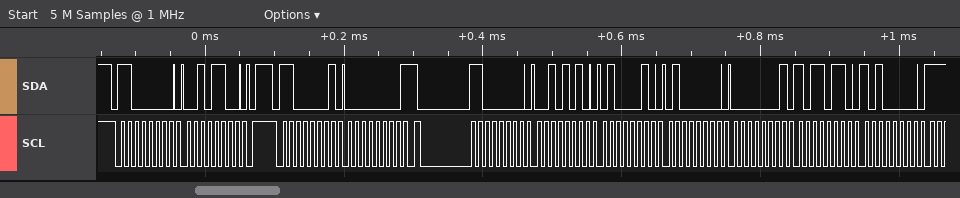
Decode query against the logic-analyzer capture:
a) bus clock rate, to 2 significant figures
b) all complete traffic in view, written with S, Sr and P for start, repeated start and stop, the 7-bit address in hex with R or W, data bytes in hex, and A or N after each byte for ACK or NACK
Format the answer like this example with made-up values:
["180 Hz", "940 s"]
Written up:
["100 kHz", "S 60W A 2C A P S 60R A 00 N Sr 60W A 2A A 42 A 40 A 01 A B6 A A0 A"]
